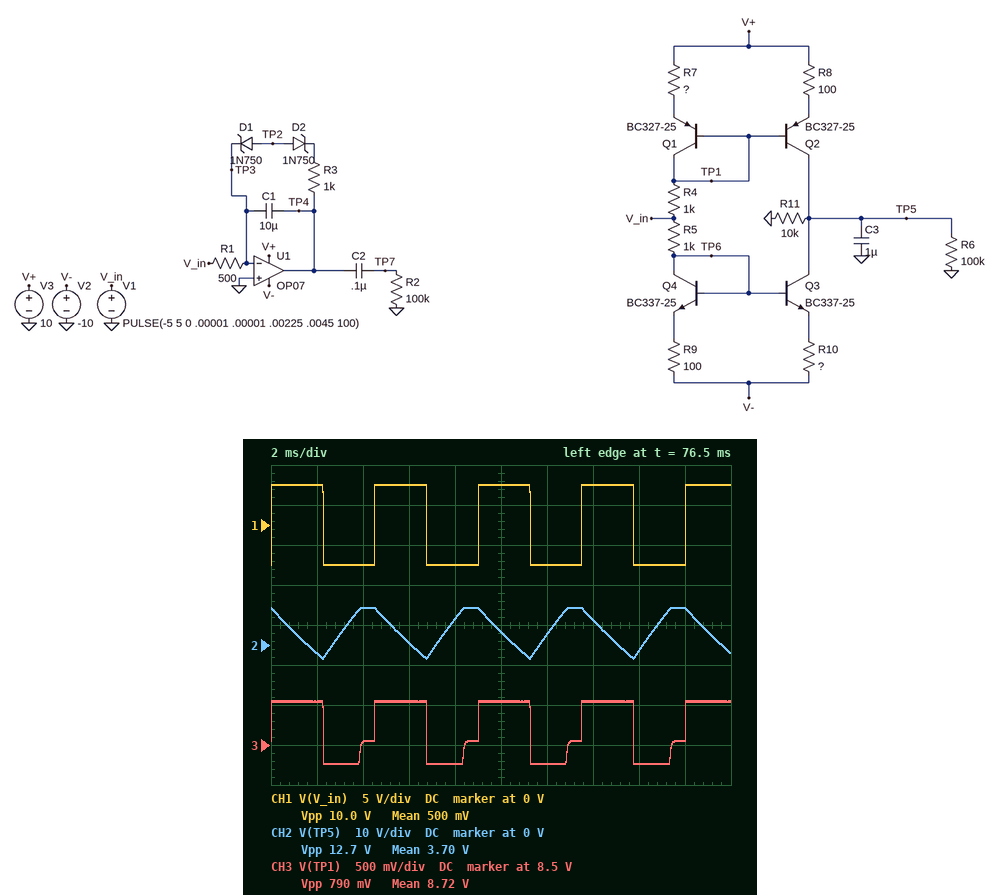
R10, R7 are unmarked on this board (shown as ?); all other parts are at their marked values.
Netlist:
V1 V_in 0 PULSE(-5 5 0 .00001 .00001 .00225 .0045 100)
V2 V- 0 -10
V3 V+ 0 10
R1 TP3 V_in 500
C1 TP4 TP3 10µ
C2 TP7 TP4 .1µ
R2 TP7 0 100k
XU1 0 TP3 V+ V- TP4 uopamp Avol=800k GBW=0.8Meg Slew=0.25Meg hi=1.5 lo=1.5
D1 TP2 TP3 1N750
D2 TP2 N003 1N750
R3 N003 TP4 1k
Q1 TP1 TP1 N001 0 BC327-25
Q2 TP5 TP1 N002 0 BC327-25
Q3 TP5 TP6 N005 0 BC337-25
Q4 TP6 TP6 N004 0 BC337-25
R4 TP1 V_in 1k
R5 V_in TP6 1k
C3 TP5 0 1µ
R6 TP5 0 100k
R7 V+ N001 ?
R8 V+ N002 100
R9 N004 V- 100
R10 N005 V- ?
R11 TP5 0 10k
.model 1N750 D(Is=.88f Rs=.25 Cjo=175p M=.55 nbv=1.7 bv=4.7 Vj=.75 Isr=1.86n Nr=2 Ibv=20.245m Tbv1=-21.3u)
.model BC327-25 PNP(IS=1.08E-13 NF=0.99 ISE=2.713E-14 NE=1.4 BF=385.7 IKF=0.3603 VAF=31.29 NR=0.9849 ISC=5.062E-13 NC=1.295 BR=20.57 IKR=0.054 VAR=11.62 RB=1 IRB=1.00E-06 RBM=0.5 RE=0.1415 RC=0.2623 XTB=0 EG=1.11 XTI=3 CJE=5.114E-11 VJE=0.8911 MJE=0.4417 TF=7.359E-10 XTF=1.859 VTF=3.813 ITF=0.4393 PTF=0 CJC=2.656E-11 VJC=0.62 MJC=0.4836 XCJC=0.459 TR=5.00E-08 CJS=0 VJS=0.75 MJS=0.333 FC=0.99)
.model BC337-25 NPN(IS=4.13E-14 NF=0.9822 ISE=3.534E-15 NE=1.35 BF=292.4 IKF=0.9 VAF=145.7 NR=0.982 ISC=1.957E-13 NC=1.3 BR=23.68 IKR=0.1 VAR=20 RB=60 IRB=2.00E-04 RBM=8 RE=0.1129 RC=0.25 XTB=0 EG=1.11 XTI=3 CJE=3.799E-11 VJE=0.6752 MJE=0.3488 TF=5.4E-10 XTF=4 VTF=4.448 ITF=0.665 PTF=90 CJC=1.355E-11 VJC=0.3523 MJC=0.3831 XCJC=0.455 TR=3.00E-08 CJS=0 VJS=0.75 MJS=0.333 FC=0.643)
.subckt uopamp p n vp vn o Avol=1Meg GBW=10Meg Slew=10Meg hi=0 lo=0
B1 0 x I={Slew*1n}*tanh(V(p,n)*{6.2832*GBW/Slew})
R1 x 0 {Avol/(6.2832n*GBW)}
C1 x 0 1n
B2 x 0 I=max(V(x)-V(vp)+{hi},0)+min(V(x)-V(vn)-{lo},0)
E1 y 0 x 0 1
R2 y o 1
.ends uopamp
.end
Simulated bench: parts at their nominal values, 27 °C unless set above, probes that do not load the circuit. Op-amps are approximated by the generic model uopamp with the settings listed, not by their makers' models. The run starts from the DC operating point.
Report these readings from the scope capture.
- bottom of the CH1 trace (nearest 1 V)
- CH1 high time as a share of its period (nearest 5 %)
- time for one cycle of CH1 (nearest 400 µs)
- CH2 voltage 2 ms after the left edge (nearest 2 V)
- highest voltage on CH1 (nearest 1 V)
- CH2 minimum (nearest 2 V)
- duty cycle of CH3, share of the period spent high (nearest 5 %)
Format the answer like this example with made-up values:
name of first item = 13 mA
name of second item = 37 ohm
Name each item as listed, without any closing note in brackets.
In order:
bottom of the CH1 trace = -5 V
CH1 high time as a share of its period = 50 %
time for one cycle of CH1 = 4.4 ms
CH2 voltage 2 ms after the left edge = -2 V
highest voltage on CH1 = 5 V
CH2 minimum = -4 V
duty cycle of CH3, share of the period spent high = 50 %
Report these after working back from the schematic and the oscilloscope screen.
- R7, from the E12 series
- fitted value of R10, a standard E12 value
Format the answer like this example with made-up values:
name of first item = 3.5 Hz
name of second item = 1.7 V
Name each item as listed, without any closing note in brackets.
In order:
R7, from the E12 series = 82 Ω
fitted value of R10, a standard E12 value = 150 Ω
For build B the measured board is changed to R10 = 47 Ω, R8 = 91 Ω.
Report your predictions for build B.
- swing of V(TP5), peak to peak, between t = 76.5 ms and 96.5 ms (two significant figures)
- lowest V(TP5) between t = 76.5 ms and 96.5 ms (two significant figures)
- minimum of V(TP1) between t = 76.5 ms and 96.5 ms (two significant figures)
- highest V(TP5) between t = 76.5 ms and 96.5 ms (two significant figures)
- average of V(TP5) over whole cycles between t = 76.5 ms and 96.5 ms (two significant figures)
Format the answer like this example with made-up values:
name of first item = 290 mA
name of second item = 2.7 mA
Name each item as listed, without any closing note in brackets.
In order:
swing of V(TP5), peak to peak, between t = 76.5 ms and 96.5 ms = 10 V
lowest V(TP5) between t = 76.5 ms and 96.5 ms = -9.5 V
minimum of V(TP1) between t = 76.5 ms and 96.5 ms = 8.3 V
highest V(TP5) between t = 76.5 ms and 96.5 ms = 660 mV
average of V(TP5) over whole cycles between t = 76.5 ms and 96.5 ms = -6.3 V
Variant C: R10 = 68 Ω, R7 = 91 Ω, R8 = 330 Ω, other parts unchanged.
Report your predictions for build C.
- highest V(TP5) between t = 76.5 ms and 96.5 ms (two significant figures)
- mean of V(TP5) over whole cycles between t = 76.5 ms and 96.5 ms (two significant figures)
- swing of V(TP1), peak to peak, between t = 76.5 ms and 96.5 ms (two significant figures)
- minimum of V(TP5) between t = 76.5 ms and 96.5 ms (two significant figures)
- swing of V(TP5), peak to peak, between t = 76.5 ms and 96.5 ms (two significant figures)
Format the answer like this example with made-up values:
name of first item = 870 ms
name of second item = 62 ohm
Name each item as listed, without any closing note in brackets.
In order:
highest V(TP5) between t = 76.5 ms and 96.5 ms = -9.4 V
mean of V(TP5) over whole cycles between t = 76.5 ms and 96.5 ms = -9.5 V
swing of V(TP1), peak to peak, between t = 76.5 ms and 96.5 ms = 860 mV
minimum of V(TP5) between t = 76.5 ms and 96.5 ms = -9.6 V
swing of V(TP5), peak to peak, between t = 76.5 ms and 96.5 ms = 210 mV
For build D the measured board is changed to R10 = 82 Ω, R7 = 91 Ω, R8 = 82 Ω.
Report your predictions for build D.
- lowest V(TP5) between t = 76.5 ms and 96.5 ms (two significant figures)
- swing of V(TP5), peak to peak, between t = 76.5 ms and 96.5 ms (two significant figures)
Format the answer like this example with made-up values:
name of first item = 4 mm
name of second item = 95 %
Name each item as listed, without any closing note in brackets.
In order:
lowest V(TP5) between t = 76.5 ms and 96.5 ms = -9.2 V
swing of V(TP5), peak to peak, between t = 76.5 ms and 96.5 ms = 18 V
